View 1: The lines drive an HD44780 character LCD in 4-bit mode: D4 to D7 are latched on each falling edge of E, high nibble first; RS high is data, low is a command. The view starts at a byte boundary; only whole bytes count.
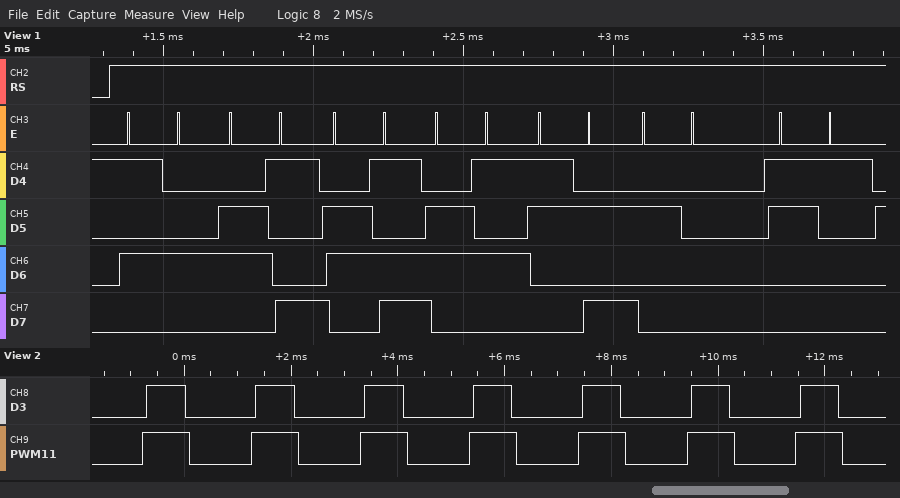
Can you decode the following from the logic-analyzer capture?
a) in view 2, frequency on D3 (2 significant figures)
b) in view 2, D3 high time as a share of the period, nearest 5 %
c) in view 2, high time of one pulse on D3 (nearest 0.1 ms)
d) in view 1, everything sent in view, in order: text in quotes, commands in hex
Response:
490 Hz
35 %
0.7 ms
"Time: 1"
